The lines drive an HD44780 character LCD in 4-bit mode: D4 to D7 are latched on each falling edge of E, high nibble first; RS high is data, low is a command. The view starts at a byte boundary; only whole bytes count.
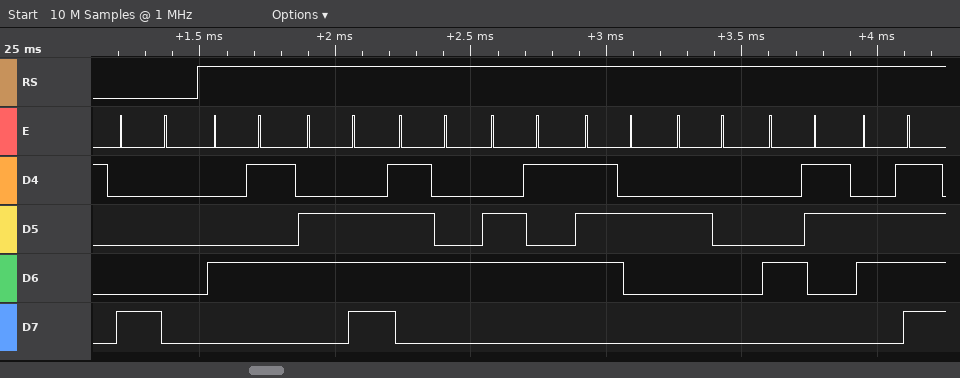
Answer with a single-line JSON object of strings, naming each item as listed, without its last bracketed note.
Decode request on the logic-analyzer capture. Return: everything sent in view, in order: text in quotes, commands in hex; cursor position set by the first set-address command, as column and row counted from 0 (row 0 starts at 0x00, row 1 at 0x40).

{"everything sent in view, in order: text in quotes, commands in hex": "0x80 \"Enter Co\"", "cursor position set by the first set-address command, as column and row counted from 0": "column 0, row 0"}
